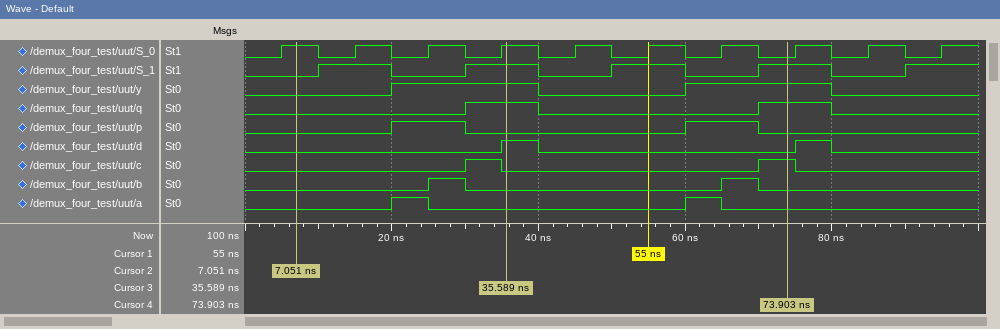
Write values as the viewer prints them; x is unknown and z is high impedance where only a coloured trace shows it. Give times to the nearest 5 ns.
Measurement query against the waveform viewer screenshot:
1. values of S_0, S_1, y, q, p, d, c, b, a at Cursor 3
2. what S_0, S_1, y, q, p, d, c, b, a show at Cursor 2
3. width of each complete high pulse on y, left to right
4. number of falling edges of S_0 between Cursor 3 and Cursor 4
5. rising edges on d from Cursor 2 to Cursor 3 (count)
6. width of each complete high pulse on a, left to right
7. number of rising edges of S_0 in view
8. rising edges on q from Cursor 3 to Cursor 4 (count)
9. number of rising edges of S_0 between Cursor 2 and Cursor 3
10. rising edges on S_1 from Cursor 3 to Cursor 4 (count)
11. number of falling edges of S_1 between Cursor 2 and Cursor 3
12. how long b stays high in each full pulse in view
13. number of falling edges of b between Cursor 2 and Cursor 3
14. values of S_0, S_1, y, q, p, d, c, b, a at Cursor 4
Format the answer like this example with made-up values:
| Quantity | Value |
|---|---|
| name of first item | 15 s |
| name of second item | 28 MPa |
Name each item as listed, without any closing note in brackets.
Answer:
| Quantity | Value |
|---|---|
| values of S_0, S_1, y, q, p, d, c, b, a at Cursor 3 | S_0=1, S_1=1, y=1, q=1, p=0, d=1, c=0, b=0, a=0 |
| what S_0, S_1, y, q, p, d, c, b, a show at Cursor 2 | S_0=1, S_1=0, y=0, q=0, p=0, d=0, c=0, b=0, a=0 |
| width of each complete high pulse on y, left to right | 20 ns, 20 ns |
| number of falling edges of S_0 between Cursor 3 and Cursor 4 | 4 |
| rising edges on d from Cursor 2 to Cursor 3 | 1 |
| width of each complete high pulse on a, left to right | 5 ns, 5 ns |
| number of rising edges of S_0 in view | 10 |
| rising edges on q from Cursor 3 to Cursor 4 | 1 |
| number of rising edges of S_0 between Cursor 2 and Cursor 3 | 3 |
| rising edges on S_1 from Cursor 3 to Cursor 4 | 2 |
| number of falling edges of S_1 between Cursor 2 and Cursor 3 | 1 |
| how long b stays high in each full pulse in view | 5 ns, 5 ns |
| number of falling edges of b between Cursor 2 and Cursor 3 | 1 |
| values of S_0, S_1, y, q, p, d, c, b, a at Cursor 4 | S_0=0, S_1=1, y=1, q=1, p=0, d=0, c=1, b=0, a=0 |
